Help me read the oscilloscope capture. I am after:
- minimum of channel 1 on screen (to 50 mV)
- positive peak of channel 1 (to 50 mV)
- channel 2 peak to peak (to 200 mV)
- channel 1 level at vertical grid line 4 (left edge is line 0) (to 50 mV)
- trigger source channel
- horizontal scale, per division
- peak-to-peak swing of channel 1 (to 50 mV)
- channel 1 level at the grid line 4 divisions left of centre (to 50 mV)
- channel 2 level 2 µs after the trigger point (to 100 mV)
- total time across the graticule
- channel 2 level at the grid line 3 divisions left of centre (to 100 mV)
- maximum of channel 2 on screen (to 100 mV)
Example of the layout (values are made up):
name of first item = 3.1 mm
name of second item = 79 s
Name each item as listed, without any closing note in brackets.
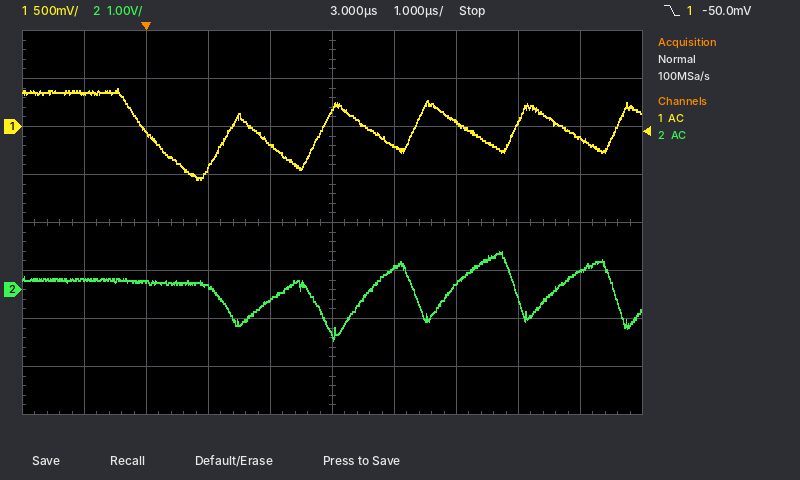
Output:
minimum of channel 1 on screen = -550 mV
positive peak of channel 1 = 400 mV
channel 2 peak to peak = 1.8 V
channel 1 level at vertical grid line 4 (left edge is line 0) = -200 mV
trigger source channel = channel 1
horizontal scale, per division = 1 µs
peak-to-peak swing of channel 1 = 950 mV
channel 1 level at the grid line 4 divisions left of centre = 350 mV
channel 2 level 2 µs after the trigger point = -200 mV
total time across the graticule = 10 µs
channel 2 level at the grid line 3 divisions left of centre = 200 mV
maximum of channel 2 on screen = 800 mV
